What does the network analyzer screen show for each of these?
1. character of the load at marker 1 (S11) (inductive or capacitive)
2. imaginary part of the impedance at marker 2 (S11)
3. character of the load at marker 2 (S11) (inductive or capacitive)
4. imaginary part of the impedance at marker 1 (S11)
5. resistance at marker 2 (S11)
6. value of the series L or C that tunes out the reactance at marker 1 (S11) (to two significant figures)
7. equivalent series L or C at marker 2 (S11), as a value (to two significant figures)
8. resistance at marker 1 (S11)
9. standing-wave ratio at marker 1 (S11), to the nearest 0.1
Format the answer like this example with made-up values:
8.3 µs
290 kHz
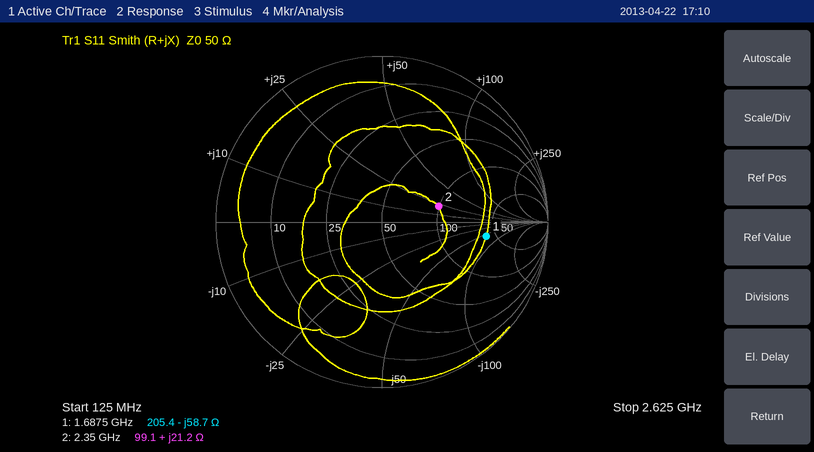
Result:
capacitive
+21.2 Ω
inductive
-58.7 Ω
99.1 Ω
5.5 nH
1.4 nH
205.4 Ω
4.5
